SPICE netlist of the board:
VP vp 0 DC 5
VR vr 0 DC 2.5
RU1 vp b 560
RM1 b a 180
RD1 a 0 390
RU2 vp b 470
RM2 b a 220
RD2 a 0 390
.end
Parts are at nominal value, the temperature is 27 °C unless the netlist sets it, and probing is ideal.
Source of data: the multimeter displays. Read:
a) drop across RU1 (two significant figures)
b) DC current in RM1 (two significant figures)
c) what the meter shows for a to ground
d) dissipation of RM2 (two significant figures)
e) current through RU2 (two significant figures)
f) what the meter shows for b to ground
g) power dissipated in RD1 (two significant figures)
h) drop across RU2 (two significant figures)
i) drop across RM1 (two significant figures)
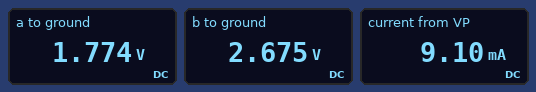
2.3 V
5.0 mA
1.774 V
3.7 mW
4.9 mA
2.675 V
8.1 mW
2.3 V
900 mV
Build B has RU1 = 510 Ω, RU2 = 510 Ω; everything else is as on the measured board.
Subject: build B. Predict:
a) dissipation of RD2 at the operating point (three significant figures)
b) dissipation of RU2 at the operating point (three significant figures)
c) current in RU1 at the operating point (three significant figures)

8.09 mW
10.6 mW
4.55 mA
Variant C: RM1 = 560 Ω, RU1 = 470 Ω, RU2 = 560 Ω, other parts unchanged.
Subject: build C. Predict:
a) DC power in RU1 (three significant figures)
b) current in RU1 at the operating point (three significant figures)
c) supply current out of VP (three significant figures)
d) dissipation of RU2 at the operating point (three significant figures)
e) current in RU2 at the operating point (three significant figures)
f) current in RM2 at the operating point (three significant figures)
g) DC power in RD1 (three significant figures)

9.38 mW
4.47 mA
8.22 mA
7.87 mW
3.75 mA
5.90 mA
6.58 mW
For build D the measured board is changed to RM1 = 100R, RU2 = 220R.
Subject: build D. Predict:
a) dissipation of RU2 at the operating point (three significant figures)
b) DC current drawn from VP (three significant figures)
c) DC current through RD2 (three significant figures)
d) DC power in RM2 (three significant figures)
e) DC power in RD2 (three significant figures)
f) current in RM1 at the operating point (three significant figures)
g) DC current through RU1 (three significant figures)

15.9 mW
11.9 mA
5.93 mA
3.02 mW
13.7 mW
8.15 mA
3.34 mA
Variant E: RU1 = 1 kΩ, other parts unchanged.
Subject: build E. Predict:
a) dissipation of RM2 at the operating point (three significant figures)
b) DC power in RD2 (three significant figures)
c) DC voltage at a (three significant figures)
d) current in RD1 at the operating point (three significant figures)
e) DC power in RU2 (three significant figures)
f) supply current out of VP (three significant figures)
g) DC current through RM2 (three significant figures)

2.96 mW
6.47 mW
1.59 V
4.07 mA
14.4 mW
8.15 mA
3.67 mA
